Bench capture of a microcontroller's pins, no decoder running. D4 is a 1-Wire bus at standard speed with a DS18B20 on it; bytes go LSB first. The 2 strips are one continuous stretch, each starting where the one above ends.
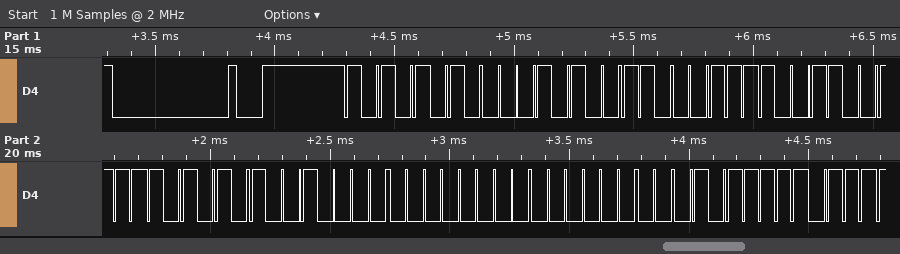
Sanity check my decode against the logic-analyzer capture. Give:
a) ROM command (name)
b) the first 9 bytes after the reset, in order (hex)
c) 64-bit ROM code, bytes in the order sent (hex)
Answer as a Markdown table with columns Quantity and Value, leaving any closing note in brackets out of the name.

| Quantity | Value |
|---|---|
| ROM command | Match ROM |
| the first 9 bytes after the reset, in order | 55 28 E3 99 57 09 00 00 FA |
| 64-bit ROM code, bytes in the order sent | 28 E3 99 57 09 00 00 FA |
